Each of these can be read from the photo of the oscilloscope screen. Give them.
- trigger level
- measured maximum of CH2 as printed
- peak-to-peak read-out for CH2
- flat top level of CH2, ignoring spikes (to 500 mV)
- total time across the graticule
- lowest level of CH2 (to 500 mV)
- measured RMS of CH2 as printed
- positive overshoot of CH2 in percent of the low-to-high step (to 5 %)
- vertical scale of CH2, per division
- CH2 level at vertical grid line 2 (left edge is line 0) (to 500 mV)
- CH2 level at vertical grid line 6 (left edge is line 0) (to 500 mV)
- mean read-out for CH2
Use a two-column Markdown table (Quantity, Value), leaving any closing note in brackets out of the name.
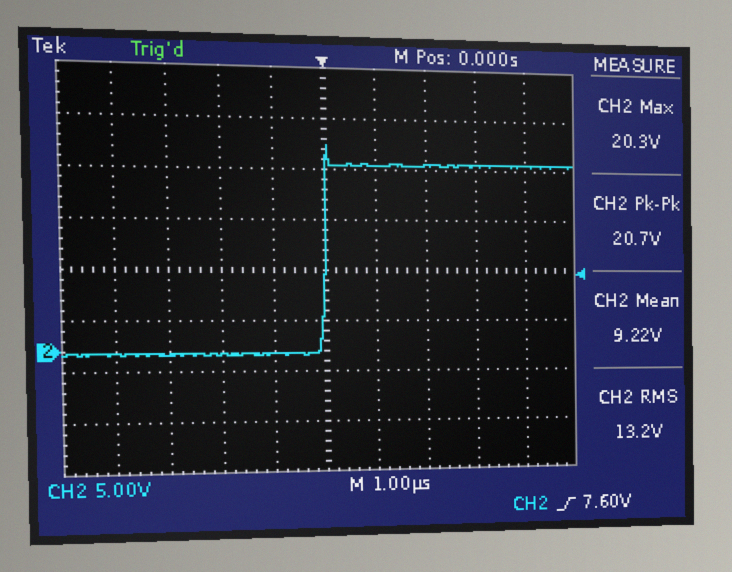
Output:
| Quantity | Value |
|---|---|
| trigger level | 7.60 V |
| measured maximum of CH2 as printed | 20.3 V |
| peak-to-peak read-out for CH2 | 20.7 V |
| flat top level of CH2, ignoring spikes | 18.5 V |
| total time across the graticule | 10 µs |
| lowest level of CH2 | -500 mV |
| measured RMS of CH2 as printed | 13.2 V |
| positive overshoot of CH2 in percent of the low-to-high step | 10 % |
| vertical scale of CH2, per division | 5 V |
| CH2 level at vertical grid line 2 (left edge is line 0) | -500 mV |
| CH2 level at vertical grid line 6 (left edge is line 0) | 18.5 V |
| mean read-out for CH2 | 9.22 V |
